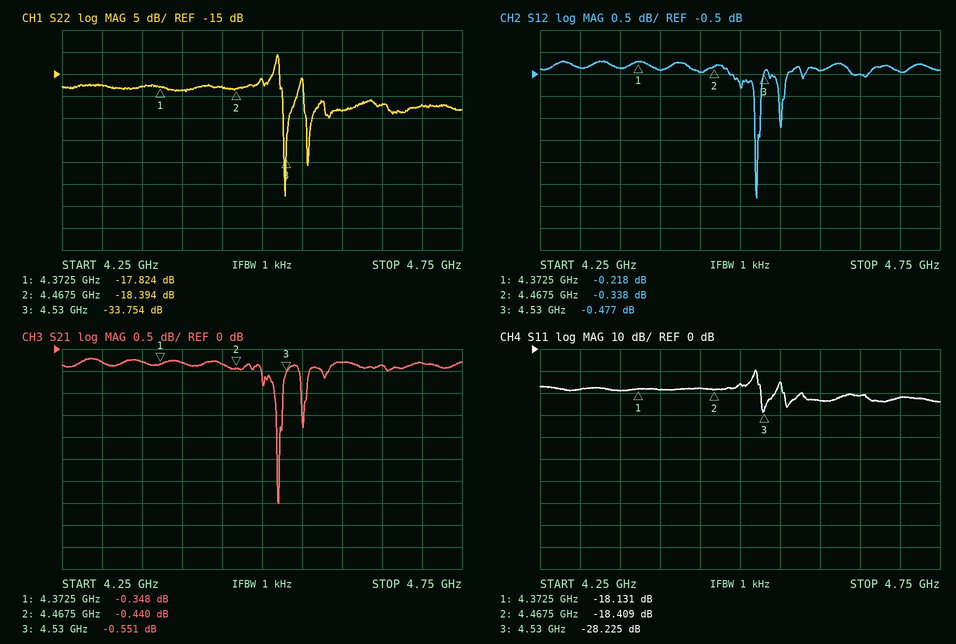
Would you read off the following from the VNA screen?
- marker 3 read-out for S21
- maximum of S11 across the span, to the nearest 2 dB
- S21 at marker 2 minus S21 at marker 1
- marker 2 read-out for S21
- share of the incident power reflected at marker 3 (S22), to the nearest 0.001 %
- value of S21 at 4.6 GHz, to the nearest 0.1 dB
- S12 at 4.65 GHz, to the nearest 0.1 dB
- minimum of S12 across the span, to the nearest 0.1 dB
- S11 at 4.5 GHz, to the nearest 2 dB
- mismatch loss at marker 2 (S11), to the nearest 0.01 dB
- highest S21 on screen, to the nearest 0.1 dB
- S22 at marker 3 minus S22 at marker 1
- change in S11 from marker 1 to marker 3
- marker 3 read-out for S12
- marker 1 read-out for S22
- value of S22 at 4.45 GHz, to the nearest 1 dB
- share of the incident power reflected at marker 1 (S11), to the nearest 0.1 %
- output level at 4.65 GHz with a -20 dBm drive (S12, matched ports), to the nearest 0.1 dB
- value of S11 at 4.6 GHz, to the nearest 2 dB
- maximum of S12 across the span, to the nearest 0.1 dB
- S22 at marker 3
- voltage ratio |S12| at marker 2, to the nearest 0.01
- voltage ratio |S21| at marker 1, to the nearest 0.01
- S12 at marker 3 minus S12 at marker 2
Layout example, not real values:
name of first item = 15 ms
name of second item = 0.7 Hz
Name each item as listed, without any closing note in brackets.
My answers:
marker 3 read-out for S21 = -0.551 dB
maximum of S11 across the span, to the nearest 2 dB = -10 dB
S21 at marker 2 minus S21 at marker 1 = -0.092 dB
marker 2 read-out for S21 = -0.440 dB
share of the incident power reflected at marker 3 (S22), to the nearest 0.001 % = 0.042 %
value of S21 at 4.6 GHz, to the nearest 0.1 dB = -0.3 dB
S12 at 4.65 GHz, to the nearest 0.1 dB = -0.5 dB
minimum of S12 across the span, to the nearest 0.1 dB = -3.3 dB
S11 at 4.5 GHz, to the nearest 2 dB = -16 dB
mismatch loss at marker 2 (S11), to the nearest 0.01 dB = 0.06 dB
highest S21 on screen, to the nearest 0.1 dB = -0.2 dB
S22 at marker 3 minus S22 at marker 1 = -15.930 dB
change in S11 from marker 1 to marker 3 = -10.094 dB
marker 3 read-out for S12 = -0.477 dB
marker 1 read-out for S22 = -17.824 dB
value of S22 at 4.45 GHz, to the nearest 1 dB = -18 dB
share of the incident power reflected at marker 1 (S11), to the nearest 0.1 % = 1.5 %
output level at 4.65 GHz with a -20 dBm drive (S12, matched ports), to the nearest 0.1 dB = -20.5 dBm
value of S11 at 4.6 GHz, to the nearest 2 dB = -24 dB
maximum of S12 across the span, to the nearest 0.1 dB = -0.2 dB
S22 at marker 3 = -33.754 dB
voltage ratio |S12| at marker 2, to the nearest 0.01 = 0.96
voltage ratio |S21| at marker 1, to the nearest 0.01 = 0.96
S12 at marker 3 minus S12 at marker 2 = -0.139 dB
